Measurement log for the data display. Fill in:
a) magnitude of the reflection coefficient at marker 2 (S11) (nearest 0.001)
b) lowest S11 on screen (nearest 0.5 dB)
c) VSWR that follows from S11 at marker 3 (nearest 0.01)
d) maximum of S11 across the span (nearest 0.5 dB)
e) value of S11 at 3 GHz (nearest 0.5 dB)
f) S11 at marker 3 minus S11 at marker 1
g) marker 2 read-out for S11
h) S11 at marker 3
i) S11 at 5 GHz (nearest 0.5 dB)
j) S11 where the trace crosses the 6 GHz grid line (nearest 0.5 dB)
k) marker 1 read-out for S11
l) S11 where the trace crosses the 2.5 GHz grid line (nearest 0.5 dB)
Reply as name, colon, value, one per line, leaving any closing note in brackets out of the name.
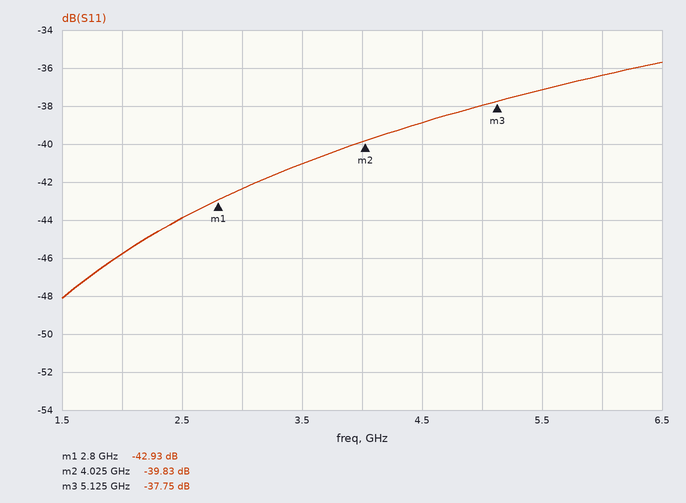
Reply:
magnitude of the reflection coefficient at marker 2 (S11): 0.010
lowest S11 on screen: -48.0 dB
VSWR that follows from S11 at marker 3: 1.03
maximum of S11 across the span: -35.5 dB
value of S11 at 3 GHz: -42.5 dB
S11 at marker 3 minus S11 at marker 1: 5.18 dB
marker 2 read-out for S11: -39.83 dB
S11 at marker 3: -37.75 dB
S11 at 5 GHz: -38.0 dB
S11 where the trace crosses the 6 GHz grid line: -36.5 dB
marker 1 read-out for S11: -42.93 dB
S11 where the trace crosses the 2.5 GHz grid line: -44.0 dB
